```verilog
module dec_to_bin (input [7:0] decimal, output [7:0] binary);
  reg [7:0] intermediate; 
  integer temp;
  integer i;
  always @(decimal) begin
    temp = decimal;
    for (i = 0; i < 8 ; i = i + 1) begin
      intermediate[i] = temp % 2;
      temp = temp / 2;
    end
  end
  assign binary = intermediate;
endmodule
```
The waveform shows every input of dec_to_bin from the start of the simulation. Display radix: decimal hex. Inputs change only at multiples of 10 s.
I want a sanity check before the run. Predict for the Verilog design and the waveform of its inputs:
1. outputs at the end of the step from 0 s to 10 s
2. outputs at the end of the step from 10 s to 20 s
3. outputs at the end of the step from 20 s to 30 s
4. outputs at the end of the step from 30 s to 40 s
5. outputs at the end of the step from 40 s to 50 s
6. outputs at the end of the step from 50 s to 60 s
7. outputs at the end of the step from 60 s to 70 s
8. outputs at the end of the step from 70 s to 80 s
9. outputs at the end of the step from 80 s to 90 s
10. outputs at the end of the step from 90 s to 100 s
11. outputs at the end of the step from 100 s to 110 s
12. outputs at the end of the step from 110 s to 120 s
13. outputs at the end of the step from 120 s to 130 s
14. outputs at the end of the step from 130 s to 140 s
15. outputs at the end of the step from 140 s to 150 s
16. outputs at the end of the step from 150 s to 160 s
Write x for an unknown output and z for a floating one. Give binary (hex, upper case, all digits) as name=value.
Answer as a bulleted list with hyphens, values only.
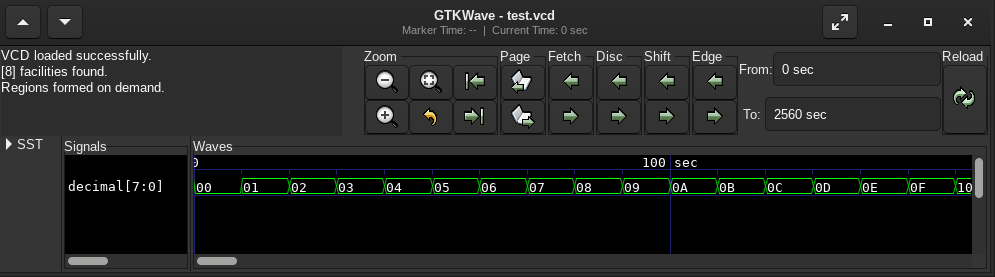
- binary=00
- binary=01
- binary=02
- binary=03
- binary=04
- binary=05
- binary=06
- binary=07
- binary=08
- binary=09
- binary=0A
- binary=0B
- binary=0C
- binary=0D
- binary=0E
- binary=0F
